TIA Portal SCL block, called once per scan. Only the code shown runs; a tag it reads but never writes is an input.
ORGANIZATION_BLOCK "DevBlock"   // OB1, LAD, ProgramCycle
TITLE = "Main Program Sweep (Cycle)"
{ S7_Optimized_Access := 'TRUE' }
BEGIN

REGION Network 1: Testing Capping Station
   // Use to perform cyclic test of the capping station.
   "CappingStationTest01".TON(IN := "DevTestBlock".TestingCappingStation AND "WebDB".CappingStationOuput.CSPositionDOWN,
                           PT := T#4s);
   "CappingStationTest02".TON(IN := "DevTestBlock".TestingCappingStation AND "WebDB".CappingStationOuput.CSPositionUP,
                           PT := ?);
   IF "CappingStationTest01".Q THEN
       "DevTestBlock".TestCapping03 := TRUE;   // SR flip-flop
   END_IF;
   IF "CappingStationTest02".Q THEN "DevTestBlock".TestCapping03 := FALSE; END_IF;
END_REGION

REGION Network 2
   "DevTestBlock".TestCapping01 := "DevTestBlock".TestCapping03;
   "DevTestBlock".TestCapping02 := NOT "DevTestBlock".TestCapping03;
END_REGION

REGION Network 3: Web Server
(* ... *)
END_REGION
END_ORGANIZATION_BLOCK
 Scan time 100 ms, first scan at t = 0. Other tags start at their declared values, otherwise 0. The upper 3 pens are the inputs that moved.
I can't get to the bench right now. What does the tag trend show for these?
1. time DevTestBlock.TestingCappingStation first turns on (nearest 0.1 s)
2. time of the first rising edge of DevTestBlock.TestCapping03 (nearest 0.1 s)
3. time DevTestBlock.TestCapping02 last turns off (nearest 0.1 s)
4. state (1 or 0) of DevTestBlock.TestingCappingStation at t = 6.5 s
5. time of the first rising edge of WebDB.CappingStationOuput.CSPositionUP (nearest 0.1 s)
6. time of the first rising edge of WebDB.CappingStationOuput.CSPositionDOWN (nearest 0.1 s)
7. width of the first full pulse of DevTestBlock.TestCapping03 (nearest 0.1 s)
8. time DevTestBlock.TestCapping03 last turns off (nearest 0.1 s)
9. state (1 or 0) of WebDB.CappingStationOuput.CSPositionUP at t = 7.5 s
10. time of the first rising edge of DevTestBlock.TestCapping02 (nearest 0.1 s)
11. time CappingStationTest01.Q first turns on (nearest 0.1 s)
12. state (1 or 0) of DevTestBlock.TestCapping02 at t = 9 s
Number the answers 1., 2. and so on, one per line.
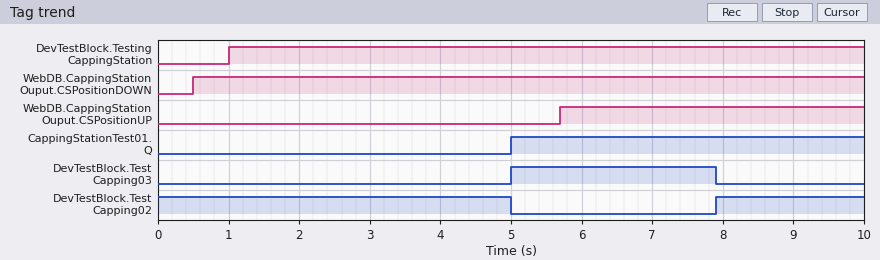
1. 1.0 s
2. 5.0 s
3. 5.0 s
4. 1
5. 5.7 s
6. 0.5 s
7. 2.9 s
8. 7.9 s
9. 1
10. 7.9 s
11. 5.0 s
12. 1
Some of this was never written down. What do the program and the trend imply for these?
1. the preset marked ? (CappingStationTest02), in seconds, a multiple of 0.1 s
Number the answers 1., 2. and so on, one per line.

1. 2.2 s
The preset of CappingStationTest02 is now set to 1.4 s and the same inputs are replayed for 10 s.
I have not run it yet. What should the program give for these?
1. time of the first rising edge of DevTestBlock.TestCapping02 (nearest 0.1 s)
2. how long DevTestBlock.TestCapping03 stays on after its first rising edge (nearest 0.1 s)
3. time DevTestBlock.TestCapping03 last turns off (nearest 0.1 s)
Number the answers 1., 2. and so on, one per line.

1. 7.1 s
2. 2.1 s
3. 7.1 s
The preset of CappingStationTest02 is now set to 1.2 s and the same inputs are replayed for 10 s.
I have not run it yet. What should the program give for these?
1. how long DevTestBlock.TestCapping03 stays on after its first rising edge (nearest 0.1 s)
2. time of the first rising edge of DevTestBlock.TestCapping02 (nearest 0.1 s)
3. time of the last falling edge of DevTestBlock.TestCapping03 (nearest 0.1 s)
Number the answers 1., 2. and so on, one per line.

1. 1.9 s
2. 6.9 s
3. 6.9 s
